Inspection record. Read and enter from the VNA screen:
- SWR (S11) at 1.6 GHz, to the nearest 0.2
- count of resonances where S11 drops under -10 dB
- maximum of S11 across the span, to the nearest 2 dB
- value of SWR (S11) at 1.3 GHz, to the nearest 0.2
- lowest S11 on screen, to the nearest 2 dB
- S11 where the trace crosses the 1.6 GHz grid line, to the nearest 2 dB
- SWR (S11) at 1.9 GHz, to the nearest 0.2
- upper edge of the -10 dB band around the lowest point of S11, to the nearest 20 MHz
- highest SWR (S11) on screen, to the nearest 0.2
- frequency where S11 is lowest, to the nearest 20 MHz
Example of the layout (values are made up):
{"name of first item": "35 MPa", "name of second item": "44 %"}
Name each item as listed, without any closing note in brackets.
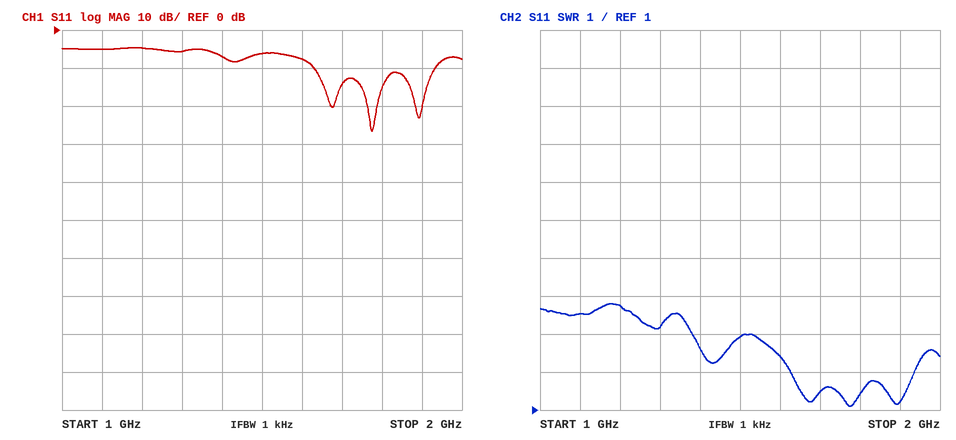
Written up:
{"SWR (S11) at 1.6 GHz, to the nearest 0.2": "2.4", "count of resonances where S11 drops under -10 dB": "3", "maximum of S11 across the span, to the nearest 2 dB": "-4 dB", "value of SWR (S11) at 1.3 GHz, to the nearest 0.2": "3.2", "lowest S11 on screen, to the nearest 2 dB": "-26 dB", "S11 where the trace crosses the 1.6 GHz grid line, to the nearest 2 dB": "-8 dB", "SWR (S11) at 1.9 GHz, to the nearest 0.2": "1.2", "upper edge of the -10 dB band around the lowest point of S11, to the nearest 20 MHz": "1.94 GHz", "highest SWR (S11) on screen, to the nearest 0.2": "3.8", "frequency where S11 is lowest, to the nearest 20 MHz": "1.78 GHz"}
